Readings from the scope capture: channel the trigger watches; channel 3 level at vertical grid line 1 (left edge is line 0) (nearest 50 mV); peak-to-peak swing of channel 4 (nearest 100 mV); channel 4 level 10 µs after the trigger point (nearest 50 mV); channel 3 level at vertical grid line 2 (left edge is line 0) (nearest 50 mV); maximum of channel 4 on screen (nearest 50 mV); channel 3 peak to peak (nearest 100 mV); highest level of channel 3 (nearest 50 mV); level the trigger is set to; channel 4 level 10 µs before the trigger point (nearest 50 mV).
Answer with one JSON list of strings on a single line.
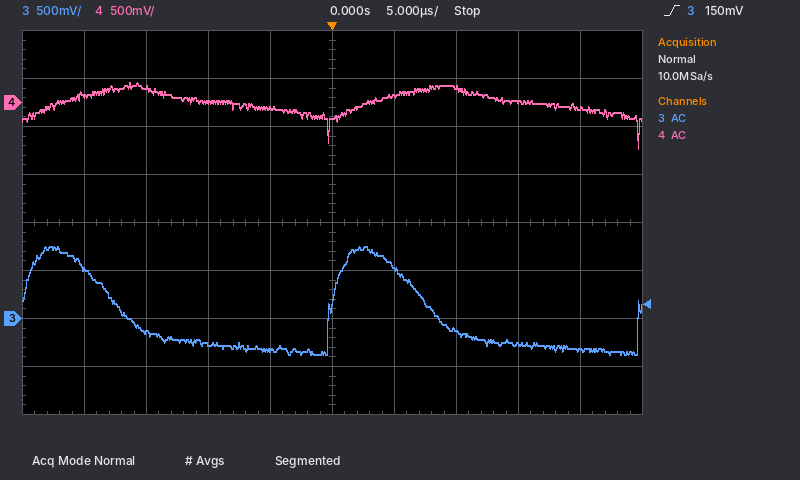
["channel 3", "550 mV", "700 mV", "150 mV", "-150 mV", "200 mV", "1.10 V", "750 mV", "150 mV", "0 mV"]
